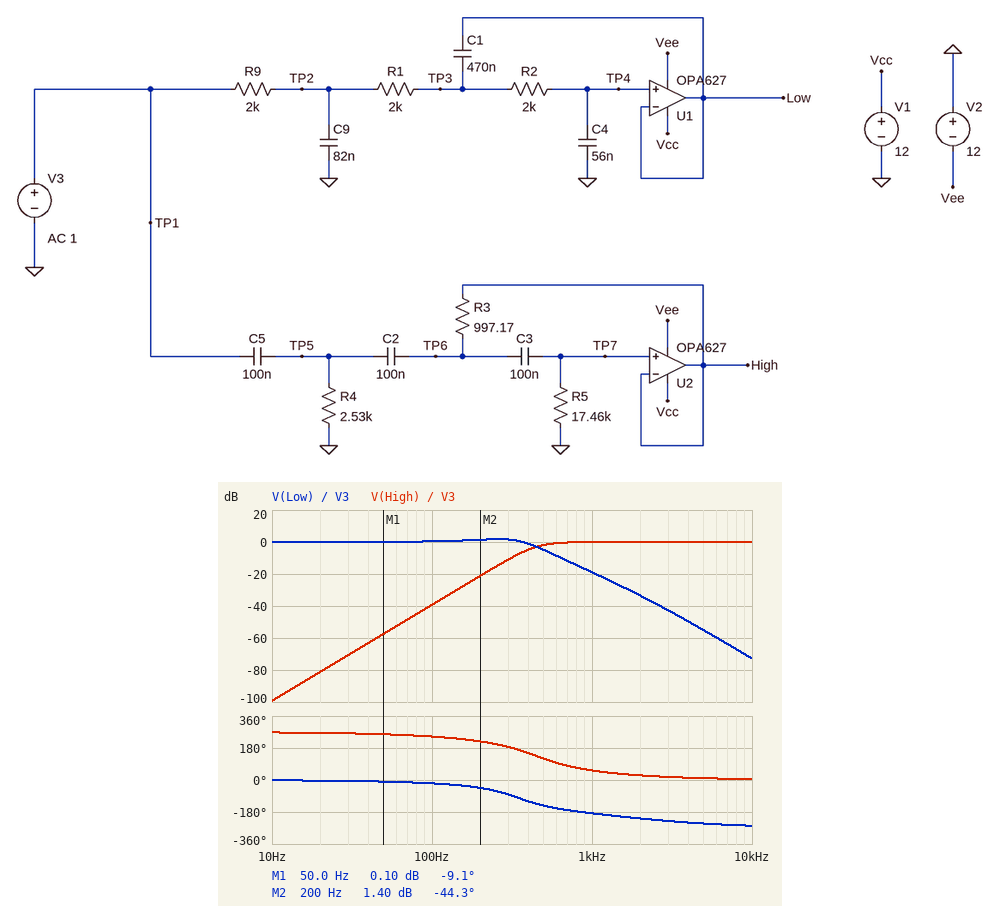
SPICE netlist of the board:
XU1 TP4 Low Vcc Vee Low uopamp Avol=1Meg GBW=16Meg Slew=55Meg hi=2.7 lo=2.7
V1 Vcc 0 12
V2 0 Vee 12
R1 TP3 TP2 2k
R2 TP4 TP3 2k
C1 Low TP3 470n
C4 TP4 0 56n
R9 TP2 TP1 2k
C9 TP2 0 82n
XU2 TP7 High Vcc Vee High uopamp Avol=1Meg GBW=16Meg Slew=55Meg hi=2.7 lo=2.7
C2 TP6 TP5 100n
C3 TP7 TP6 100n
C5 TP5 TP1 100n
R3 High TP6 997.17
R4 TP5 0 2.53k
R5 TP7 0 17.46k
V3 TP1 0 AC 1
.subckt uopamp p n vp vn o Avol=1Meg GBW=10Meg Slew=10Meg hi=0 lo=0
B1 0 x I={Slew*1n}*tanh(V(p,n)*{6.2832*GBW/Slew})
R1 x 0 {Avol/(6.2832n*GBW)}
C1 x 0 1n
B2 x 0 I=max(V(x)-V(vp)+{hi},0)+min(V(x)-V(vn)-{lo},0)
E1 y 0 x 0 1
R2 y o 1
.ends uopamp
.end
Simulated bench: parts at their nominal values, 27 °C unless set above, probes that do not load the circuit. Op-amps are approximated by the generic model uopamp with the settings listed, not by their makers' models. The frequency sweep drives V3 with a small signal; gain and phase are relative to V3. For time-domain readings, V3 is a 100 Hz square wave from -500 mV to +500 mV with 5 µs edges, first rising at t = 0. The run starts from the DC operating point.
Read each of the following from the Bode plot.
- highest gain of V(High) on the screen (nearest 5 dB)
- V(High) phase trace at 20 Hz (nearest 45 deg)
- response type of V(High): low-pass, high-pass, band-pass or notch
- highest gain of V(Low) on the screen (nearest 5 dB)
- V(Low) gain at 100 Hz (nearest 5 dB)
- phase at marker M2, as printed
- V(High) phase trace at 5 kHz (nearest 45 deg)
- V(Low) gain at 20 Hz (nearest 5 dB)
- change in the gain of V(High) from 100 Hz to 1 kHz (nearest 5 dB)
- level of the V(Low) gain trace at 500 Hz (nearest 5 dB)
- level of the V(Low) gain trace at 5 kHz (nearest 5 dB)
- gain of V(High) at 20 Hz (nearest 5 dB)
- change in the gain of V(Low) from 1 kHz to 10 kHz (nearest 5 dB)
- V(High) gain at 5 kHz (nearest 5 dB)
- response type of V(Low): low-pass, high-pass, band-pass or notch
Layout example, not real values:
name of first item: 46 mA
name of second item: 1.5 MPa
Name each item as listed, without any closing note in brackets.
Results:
highest gain of V(High) on the screen: 0 dB
V(High) phase trace at 20 Hz: 270 deg
response type of V(High): low-pass, high-pass, band-pass or notch: high-pass
highest gain of V(Low) on the screen: 0 dB
V(Low) gain at 100 Hz: 0 dB
phase at marker M2, as printed: -44.3 deg
V(High) phase trace at 5 kHz: 0 deg
V(Low) gain at 20 Hz: 0 dB
change in the gain of V(High) from 100 Hz to 1 kHz: 40 dB
level of the V(Low) gain trace at 500 Hz: -5 dB
level of the V(Low) gain trace at 5 kHz: -55 dB
gain of V(High) at 20 Hz: -80 dB
change in the gain of V(Low) from 1 kHz to 10 kHz: -55 dB
V(High) gain at 5 kHz: 0 dB
response type of V(Low): low-pass, high-pass, band-pass or notch: low-pass
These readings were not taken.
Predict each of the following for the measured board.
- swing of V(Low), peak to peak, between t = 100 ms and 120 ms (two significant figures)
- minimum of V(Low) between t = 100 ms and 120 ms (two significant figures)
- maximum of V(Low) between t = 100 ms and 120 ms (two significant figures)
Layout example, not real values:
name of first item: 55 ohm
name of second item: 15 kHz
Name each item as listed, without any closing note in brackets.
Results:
swing of V(Low), peak to peak, between t = 100 ms and 120 ms: 1.4 V
minimum of V(Low) between t = 100 ms and 120 ms: -700 mV
maximum of V(Low) between t = 100 ms and 120 ms: 700 mV
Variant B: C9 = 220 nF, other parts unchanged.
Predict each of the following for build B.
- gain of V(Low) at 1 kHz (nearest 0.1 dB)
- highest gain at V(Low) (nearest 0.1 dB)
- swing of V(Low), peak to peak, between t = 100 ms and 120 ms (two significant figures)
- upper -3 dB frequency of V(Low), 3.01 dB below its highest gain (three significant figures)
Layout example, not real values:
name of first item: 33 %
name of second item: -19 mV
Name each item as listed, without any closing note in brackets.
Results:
gain of V(Low) at 1 kHz: -22.3 dB
highest gain at V(Low): 0 dB
swing of V(Low), peak to peak, between t = 100 ms and 120 ms: 1.1 V
upper -3 dB frequency of V(Low), 3.01 dB below its highest gain: 374 Hz
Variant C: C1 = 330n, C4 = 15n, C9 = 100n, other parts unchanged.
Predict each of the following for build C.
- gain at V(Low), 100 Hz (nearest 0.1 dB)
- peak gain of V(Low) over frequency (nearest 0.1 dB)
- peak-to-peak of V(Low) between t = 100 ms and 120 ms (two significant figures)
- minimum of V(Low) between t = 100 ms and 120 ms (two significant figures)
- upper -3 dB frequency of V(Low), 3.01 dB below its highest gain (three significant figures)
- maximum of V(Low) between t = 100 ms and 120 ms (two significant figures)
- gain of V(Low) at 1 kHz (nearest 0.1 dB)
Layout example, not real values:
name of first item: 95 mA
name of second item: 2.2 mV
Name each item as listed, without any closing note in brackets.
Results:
gain at V(Low), 100 Hz: 0 dB
peak gain of V(Low) over frequency: 0.7 dB
peak-to-peak of V(Low) between t = 100 ms and 120 ms: 1.3 V
minimum of V(Low) between t = 100 ms and 120 ms: -640 mV
upper -3 dB frequency of V(Low), 3.01 dB below its highest gain: 986 Hz
maximum of V(Low) between t = 100 ms and 120 ms: 640 mV
gain of V(Low) at 1 kHz: -2.5 dB
